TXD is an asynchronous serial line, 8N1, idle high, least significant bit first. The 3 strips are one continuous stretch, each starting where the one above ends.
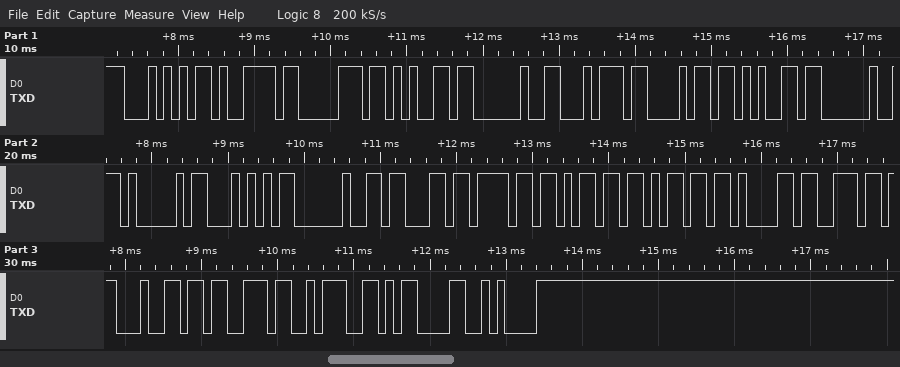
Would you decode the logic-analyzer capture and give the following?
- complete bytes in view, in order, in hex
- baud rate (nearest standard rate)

0x54 0x79 0x70 0x65 0x20 0x74 0x68 0x65 0x20 0x41 0x54 0x20 0x63 0x6F 0x6D 0x6D 0x61 0x6E 0x64 0x73 0x3A 0x0D 0x0A
9600 baud
